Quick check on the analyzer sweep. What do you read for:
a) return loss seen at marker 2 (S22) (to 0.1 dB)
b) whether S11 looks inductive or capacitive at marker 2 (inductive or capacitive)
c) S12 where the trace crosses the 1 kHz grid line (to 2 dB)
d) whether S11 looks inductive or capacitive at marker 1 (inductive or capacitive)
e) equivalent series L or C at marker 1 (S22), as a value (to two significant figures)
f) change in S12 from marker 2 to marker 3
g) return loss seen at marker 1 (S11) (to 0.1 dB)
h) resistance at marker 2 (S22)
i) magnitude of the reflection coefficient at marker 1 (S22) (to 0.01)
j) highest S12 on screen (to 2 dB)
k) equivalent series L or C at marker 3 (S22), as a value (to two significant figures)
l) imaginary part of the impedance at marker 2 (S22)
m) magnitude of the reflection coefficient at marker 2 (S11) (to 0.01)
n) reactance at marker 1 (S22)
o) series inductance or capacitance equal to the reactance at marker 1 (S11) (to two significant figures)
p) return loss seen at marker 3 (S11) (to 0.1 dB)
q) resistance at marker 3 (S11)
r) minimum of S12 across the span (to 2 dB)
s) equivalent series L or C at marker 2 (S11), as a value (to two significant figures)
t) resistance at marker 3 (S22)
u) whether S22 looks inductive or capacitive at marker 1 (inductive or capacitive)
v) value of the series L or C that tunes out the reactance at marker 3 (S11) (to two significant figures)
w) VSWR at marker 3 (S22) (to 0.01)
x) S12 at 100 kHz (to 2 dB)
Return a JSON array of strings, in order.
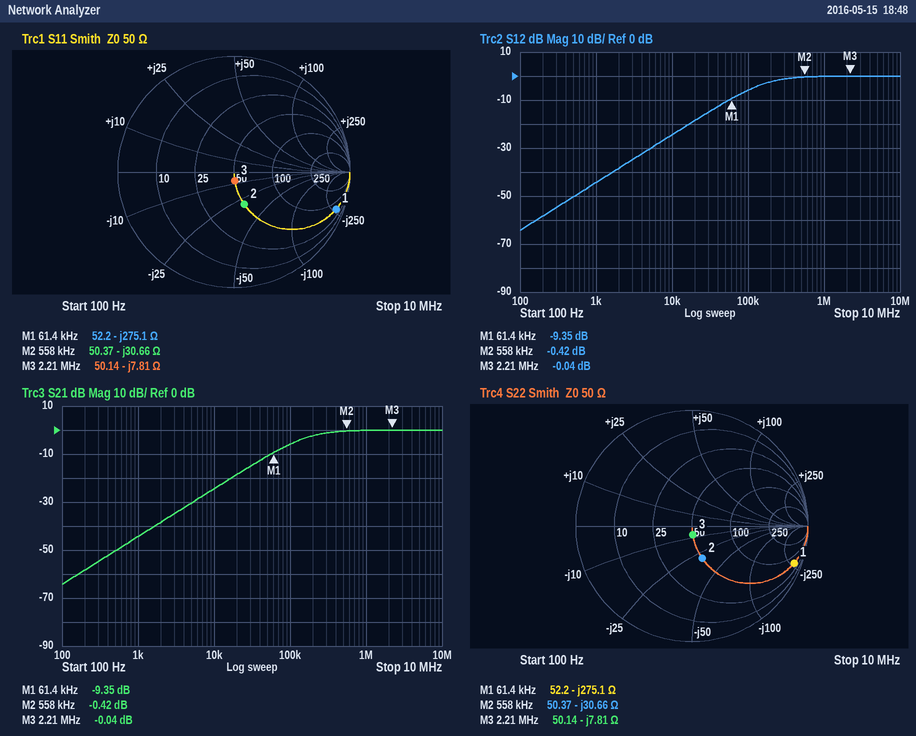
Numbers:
["10.7 dB", "capacitive", "-44 dB", "capacitive", "9.4 nF", "0.38 dB", "0.6 dB", "50.37 Ω", "0.94", "0 dB", "9.2 nF", "-30.66 Ω", "0.29", "-275.1 Ω", "9.4 nF", "22.2 dB", "50.14 Ω", "-64 dB", "9.3 nF", "50.14 Ω", "capacitive", "560 nH", "1.17", "-6 dB"]
